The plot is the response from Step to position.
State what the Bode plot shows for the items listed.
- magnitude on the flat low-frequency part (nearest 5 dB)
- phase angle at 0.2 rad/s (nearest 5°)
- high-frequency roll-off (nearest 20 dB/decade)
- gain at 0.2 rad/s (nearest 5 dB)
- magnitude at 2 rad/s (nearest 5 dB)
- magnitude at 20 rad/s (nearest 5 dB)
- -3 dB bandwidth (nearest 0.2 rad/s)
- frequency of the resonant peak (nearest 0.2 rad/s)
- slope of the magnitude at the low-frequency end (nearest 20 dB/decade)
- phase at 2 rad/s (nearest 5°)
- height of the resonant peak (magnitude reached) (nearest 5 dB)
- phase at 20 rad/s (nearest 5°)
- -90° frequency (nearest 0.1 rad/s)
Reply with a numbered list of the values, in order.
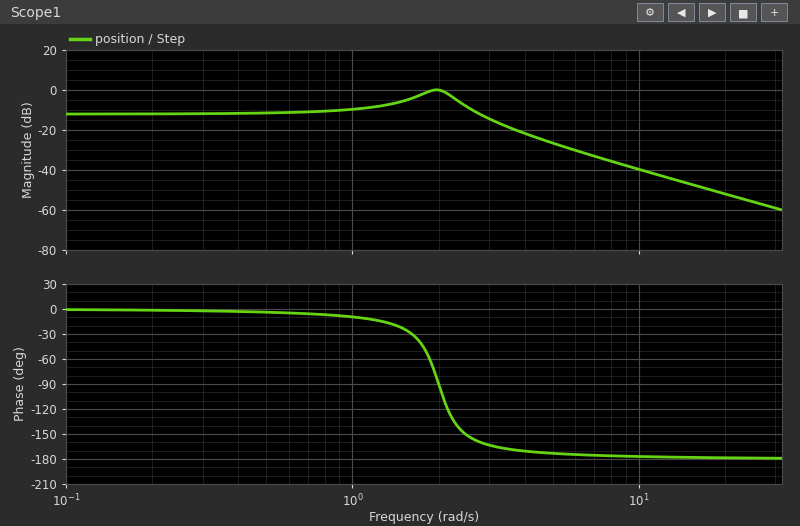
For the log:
1. -10 dB
2. 0°
3. -40 dB/decade
4. -10 dB
5. 0 dB
6. -50 dB
7. 3.0 rad/s
8. 2.0 rad/s
9. 0 dB/decade
10. -90°
11. 0 dB
12. -180°
13. 2.0 rad/s
